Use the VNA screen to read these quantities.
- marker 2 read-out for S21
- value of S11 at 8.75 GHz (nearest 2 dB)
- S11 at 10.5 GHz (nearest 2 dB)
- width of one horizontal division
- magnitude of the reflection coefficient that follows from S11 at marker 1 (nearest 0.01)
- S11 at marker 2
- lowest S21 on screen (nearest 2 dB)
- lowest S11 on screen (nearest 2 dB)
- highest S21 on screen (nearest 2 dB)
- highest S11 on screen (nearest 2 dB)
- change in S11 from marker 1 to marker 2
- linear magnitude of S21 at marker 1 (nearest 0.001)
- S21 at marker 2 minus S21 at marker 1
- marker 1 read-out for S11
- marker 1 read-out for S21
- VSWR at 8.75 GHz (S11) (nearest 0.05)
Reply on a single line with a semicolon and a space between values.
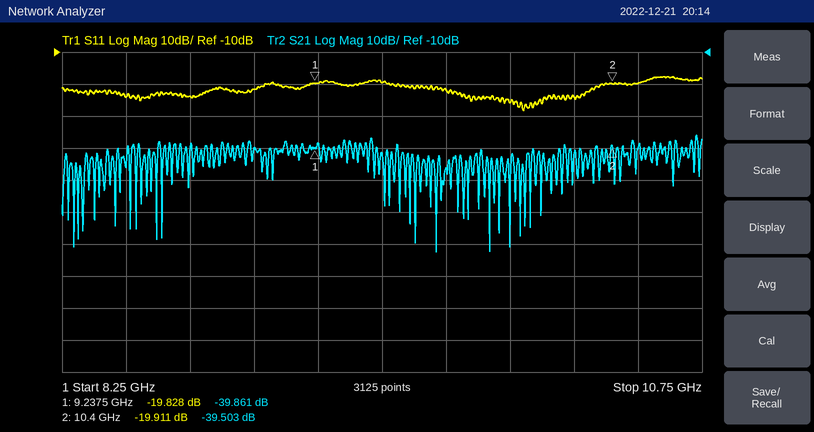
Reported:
-39.503 dB; -24 dB; -20 dB; 250 MHz; 0.10; -19.911 dB; -72 dB; -28 dB; -36 dB; -18 dB; -0.083 dB; 0.010; 0.358 dB; -19.828 dB; -39.861 dB; 1.15
